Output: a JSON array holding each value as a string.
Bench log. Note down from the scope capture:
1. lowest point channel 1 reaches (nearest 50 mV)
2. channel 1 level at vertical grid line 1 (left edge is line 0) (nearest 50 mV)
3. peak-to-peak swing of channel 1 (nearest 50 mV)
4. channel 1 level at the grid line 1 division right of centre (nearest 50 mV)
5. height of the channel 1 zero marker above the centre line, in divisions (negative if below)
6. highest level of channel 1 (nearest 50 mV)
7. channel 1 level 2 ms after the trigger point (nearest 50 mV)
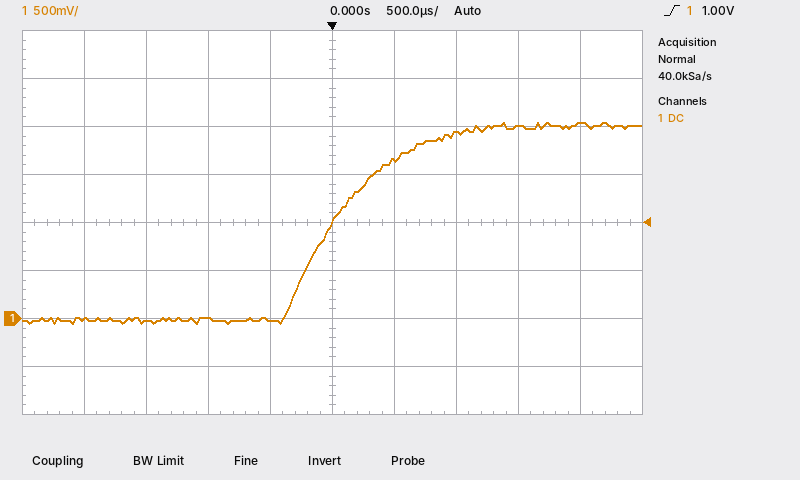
["-50 mV", "0 mV", "2.10 V", "1.65 V", "-2.0 div", "2.05 V", "2.05 V"]
